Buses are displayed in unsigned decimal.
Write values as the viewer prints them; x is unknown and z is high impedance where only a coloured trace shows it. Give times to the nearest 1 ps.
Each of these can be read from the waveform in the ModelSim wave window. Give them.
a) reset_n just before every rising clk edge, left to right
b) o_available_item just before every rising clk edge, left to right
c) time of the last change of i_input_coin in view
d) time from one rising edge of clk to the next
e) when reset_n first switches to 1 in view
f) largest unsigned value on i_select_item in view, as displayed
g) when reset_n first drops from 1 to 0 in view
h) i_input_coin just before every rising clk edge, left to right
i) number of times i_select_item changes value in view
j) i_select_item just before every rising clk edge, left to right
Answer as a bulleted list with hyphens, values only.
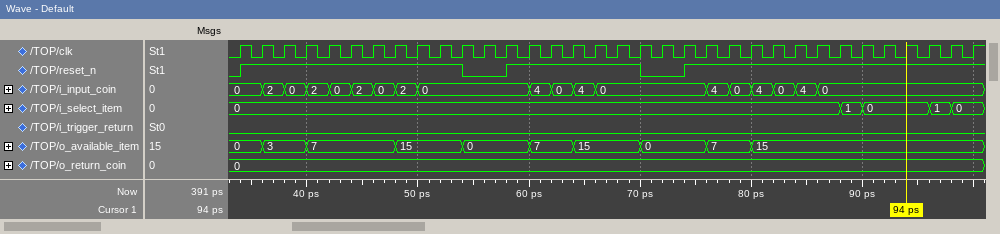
- 0 1 1 1 1 1 1 1 1 1 1 0 0 1 1 1 1 1 1 0 0 1 1 1 1 1 1 1 1 1 1 1 1 1
- 0, 0, 3, 3, 7, 7, 7, 7, 15, 15, 15, 0, 0, 0, 7, 7, 15, 15, 15, 0, 0, 0, 7, 7, 15, 15, 15, 15, 15, 15, 15, 15, 15, 15
- 86 ps
- 2 ps
- 34 ps
- 1
- 54 ps
- 0, 0, 2, 0, 2, 0, 2, 0, 2, 0, 0, 0, 0, 0, 4, 0, 4, 0, 0, 0, 0, 0, 4, 0, 4, 0, 4, 0, 0, 0, 0, 0, 0, 0
- 4
- 0, 0, 0, 0, 0, 0, 0, 0, 0, 0, 0, 0, 0, 0, 0, 0, 0, 0, 0, 0, 0, 0, 0, 0, 0, 0, 0, 0, 1, 0, 0, 0, 1, 0
